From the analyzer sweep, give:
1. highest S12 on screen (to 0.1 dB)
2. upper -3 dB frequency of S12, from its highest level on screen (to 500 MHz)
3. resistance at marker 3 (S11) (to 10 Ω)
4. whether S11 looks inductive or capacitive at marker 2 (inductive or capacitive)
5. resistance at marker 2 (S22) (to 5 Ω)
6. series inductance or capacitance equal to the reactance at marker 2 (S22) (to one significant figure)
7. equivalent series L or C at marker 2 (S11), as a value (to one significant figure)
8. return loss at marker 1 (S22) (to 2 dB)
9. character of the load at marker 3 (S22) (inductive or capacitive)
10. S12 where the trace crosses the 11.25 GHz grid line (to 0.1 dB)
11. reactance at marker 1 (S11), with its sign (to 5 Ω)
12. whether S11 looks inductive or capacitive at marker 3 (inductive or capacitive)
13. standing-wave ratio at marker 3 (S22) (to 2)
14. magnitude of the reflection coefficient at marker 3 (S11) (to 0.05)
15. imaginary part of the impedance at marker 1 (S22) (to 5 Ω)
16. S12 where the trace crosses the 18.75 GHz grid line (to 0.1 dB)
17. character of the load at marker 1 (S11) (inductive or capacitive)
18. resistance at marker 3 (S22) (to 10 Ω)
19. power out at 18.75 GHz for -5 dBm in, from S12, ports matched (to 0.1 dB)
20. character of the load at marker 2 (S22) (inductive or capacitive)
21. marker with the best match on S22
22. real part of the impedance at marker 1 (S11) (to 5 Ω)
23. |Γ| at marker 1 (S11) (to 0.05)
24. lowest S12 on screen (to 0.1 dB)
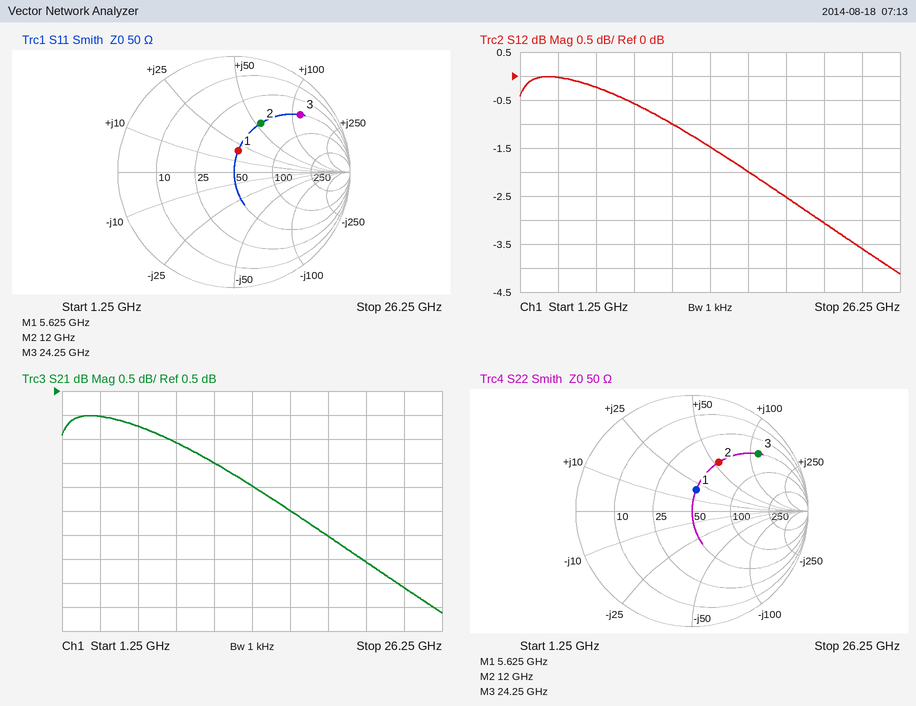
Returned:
0.0 dB
21.0 GHz
50 Ω
inductive
50 Ω
700 pH
700 pH
14 dB
inductive
-1.0 dB
+20 Ω
inductive
8
0.75
+20 Ω
-2.5 dB
inductive
50 Ω
-7.5 dBm
inductive
marker 1
50 Ω
0.20
-4.1 dB
